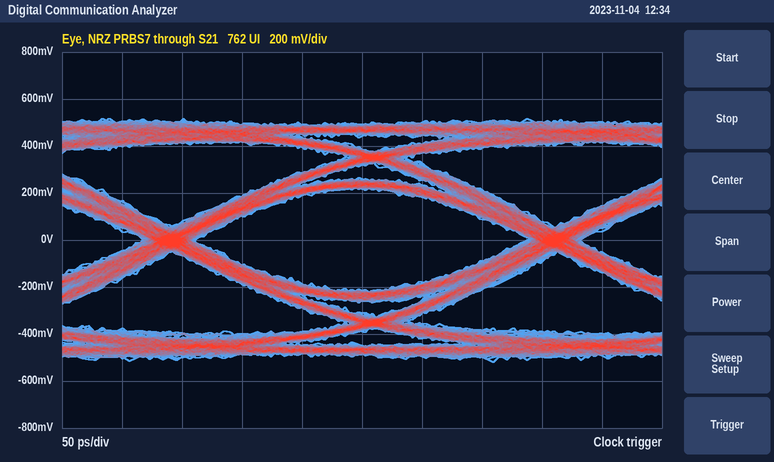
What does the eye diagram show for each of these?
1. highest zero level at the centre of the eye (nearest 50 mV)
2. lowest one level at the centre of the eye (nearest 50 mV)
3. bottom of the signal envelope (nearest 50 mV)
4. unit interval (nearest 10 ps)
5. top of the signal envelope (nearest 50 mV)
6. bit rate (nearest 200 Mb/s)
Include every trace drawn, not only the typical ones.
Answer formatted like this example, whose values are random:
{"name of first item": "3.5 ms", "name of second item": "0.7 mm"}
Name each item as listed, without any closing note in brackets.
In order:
{"highest zero level at the centre of the eye": "-200 mV", "lowest one level at the centre of the eye": "200 mV", "bottom of the signal envelope": "-500 mV", "unit interval": "320 ps", "top of the signal envelope": "500 mV", "bit rate": "3.2 Gb/s"}
